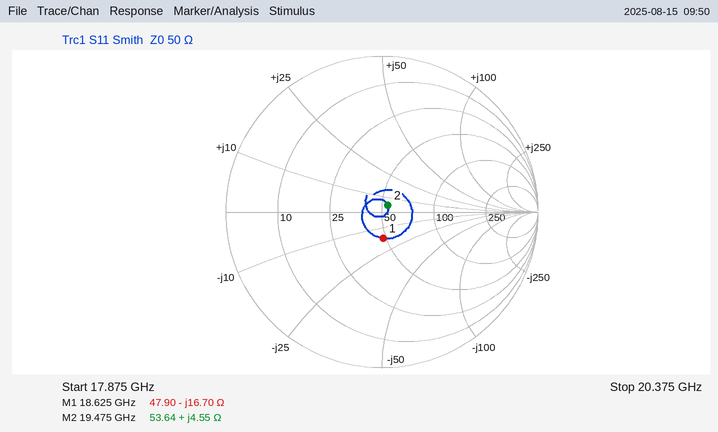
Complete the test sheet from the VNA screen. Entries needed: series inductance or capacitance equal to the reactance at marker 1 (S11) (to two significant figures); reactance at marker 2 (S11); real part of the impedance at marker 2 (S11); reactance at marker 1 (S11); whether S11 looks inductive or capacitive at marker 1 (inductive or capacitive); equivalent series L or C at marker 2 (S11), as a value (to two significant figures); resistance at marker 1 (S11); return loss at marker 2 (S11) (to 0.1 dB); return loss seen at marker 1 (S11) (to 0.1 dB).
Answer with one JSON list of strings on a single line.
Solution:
["510 fF", "+4.55 Ω", "53.64 Ω", "-16.70 Ω", "capacitive", "37 pH", "47.90 Ω", "25.0 dB", "15.4 dB"]
